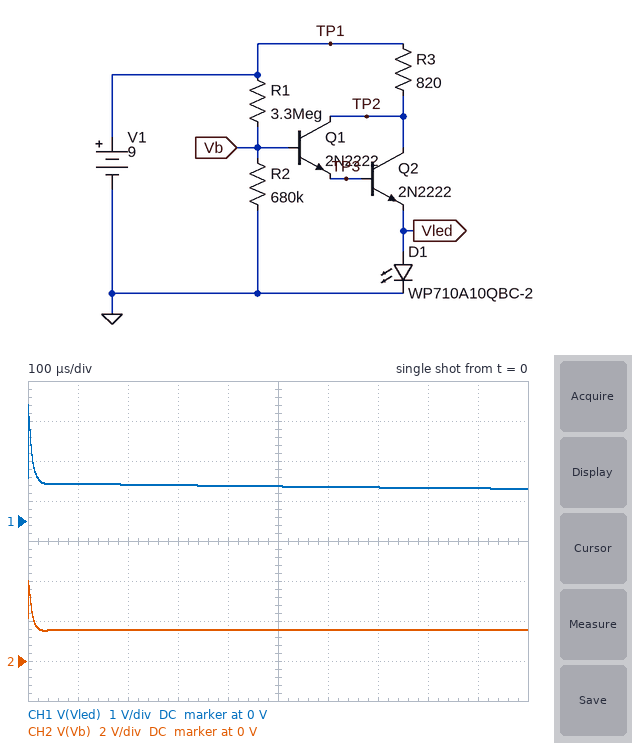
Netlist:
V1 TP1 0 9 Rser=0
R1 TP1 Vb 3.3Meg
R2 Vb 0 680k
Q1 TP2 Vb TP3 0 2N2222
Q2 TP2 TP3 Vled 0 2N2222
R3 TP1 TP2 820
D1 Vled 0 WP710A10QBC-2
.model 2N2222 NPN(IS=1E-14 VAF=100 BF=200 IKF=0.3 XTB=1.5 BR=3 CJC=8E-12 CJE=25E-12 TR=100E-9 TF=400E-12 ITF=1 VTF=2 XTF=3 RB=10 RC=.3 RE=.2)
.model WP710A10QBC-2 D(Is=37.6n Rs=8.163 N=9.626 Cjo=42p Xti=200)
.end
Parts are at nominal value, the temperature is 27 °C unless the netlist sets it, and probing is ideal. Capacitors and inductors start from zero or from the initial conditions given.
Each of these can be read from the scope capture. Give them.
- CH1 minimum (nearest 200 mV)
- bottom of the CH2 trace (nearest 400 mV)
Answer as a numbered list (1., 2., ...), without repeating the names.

1. 800 mV
2. 1.6 V
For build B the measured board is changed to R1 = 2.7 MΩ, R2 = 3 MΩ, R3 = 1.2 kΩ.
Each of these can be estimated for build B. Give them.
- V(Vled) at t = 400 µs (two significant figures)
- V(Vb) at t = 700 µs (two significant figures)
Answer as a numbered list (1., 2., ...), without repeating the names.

1. 2.9 V
2. 4.2 V
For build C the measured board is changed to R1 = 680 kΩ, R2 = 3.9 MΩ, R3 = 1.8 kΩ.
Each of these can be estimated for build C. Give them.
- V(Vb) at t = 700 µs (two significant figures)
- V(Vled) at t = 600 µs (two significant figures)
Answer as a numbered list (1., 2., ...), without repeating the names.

1. 4.1 V
2. 2.8 V
